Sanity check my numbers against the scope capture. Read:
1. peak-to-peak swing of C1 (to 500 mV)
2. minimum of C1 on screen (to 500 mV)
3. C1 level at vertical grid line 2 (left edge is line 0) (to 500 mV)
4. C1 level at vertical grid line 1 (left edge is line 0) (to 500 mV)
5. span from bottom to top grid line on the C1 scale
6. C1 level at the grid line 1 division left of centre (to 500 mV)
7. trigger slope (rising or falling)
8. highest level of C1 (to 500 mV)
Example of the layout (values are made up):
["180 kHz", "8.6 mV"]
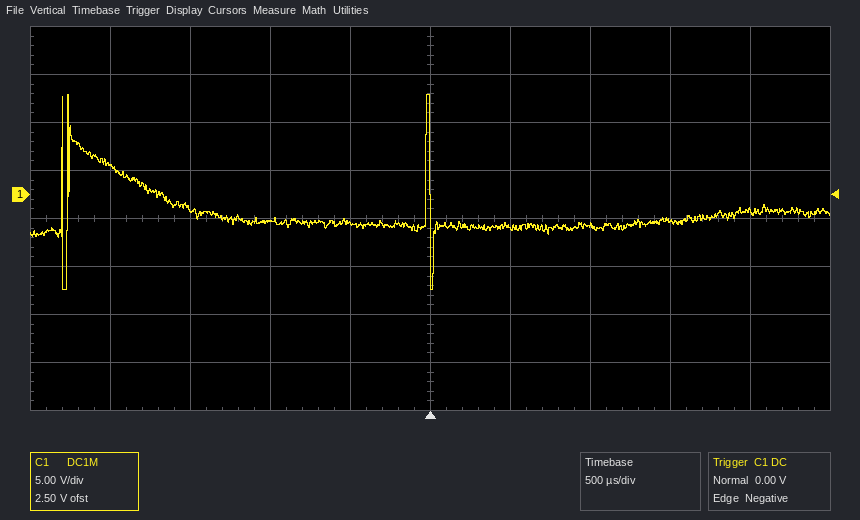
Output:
["20.5 V", "-10.0 V", "-1.5 V", "3.0 V", "40 V", "-3.0 V", "falling", "10.5 V"]
